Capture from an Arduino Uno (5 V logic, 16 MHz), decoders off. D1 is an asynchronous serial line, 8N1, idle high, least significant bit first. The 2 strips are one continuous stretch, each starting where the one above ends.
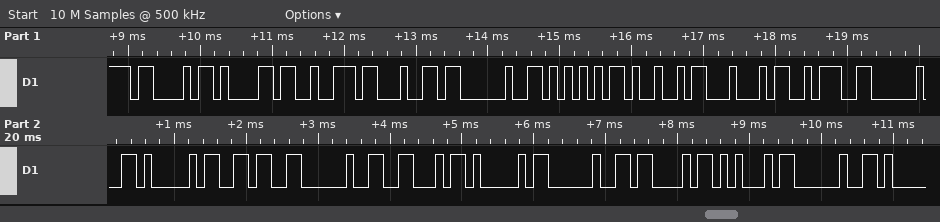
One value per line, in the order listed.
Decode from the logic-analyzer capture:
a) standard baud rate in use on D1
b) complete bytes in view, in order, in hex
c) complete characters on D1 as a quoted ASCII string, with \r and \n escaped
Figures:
9600 baud
43 61 72 64 20 55 49 44 3A 20 41 36 20 46 41 20 43 45 20
"Card UID: A6 FA CE "
